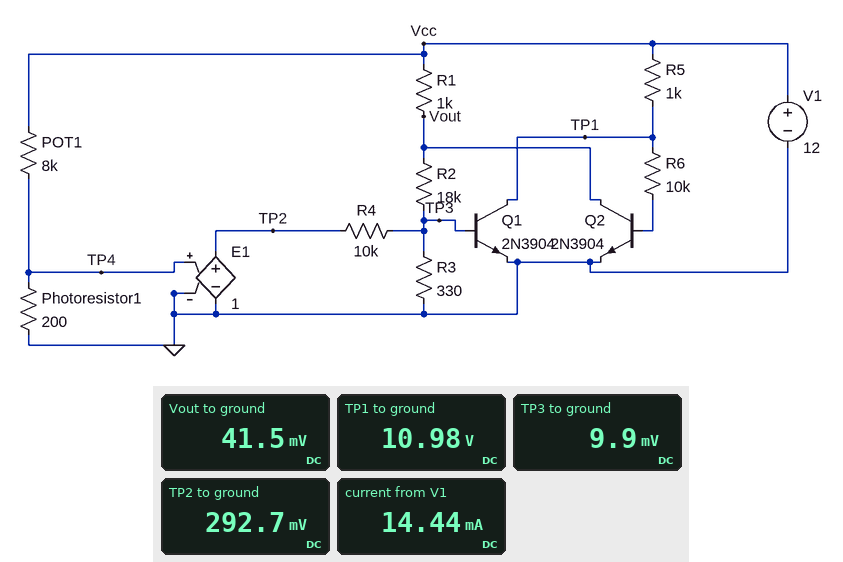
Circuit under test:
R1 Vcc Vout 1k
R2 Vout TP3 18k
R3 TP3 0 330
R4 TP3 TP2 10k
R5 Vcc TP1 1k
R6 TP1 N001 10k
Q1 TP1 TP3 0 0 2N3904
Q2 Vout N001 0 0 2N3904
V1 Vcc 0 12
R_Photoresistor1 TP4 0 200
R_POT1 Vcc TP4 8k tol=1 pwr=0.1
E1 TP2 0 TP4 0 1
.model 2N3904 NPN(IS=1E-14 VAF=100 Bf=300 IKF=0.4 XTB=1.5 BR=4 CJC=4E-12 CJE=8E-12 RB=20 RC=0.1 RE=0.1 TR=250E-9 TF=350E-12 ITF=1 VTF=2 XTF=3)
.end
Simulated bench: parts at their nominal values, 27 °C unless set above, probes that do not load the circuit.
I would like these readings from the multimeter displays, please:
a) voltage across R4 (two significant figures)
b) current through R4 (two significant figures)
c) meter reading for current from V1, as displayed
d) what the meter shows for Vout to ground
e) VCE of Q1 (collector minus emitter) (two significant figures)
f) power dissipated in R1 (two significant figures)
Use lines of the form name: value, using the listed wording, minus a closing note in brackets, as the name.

voltage across R4: 280 mV
current through R4: 28 µA
meter reading for current from V1, as displayed: 14.44 mA
what the meter shows for Vout to ground: 41.5 mV
VCE of Q1 (collector minus emitter): 11 V
power dissipated in R1: 140 mW
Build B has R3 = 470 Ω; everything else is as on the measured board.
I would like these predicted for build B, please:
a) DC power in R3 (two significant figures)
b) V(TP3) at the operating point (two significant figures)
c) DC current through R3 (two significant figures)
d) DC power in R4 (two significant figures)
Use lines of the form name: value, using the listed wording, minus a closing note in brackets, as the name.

DC power in R3: 410 nW
V(TP3) at the operating point: 14 mV
DC current through R3: 29 µA
DC power in R4: 7.8 µW
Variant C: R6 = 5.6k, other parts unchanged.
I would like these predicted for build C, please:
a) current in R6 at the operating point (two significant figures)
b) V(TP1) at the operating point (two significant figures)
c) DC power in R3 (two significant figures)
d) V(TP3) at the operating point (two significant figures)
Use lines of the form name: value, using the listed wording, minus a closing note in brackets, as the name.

current in R6 at the operating point: 1.7 mA
V(TP1) at the operating point: 10 V
DC power in R3: 290 nW
V(TP3) at the operating point: 9.8 mV
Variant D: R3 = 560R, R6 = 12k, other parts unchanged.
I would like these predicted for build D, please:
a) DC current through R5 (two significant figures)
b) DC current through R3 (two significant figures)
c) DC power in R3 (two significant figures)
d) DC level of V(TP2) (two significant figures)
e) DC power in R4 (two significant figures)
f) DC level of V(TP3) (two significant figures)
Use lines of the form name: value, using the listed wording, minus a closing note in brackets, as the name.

DC current through R5: 870 µA
DC current through R3: 29 µA
DC power in R3: 480 nW
DC level of V(TP2): 290 mV
DC power in R4: 7.6 µW
DC level of V(TP3): 16 mV
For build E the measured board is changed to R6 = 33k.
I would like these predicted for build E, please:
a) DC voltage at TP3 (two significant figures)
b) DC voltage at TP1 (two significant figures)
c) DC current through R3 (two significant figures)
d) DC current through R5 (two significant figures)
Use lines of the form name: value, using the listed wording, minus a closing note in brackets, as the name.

DC voltage at TP3: 10 mV
DC voltage at TP1: 12 V
DC current through R3: 31 µA
DC current through R5: 330 µA
